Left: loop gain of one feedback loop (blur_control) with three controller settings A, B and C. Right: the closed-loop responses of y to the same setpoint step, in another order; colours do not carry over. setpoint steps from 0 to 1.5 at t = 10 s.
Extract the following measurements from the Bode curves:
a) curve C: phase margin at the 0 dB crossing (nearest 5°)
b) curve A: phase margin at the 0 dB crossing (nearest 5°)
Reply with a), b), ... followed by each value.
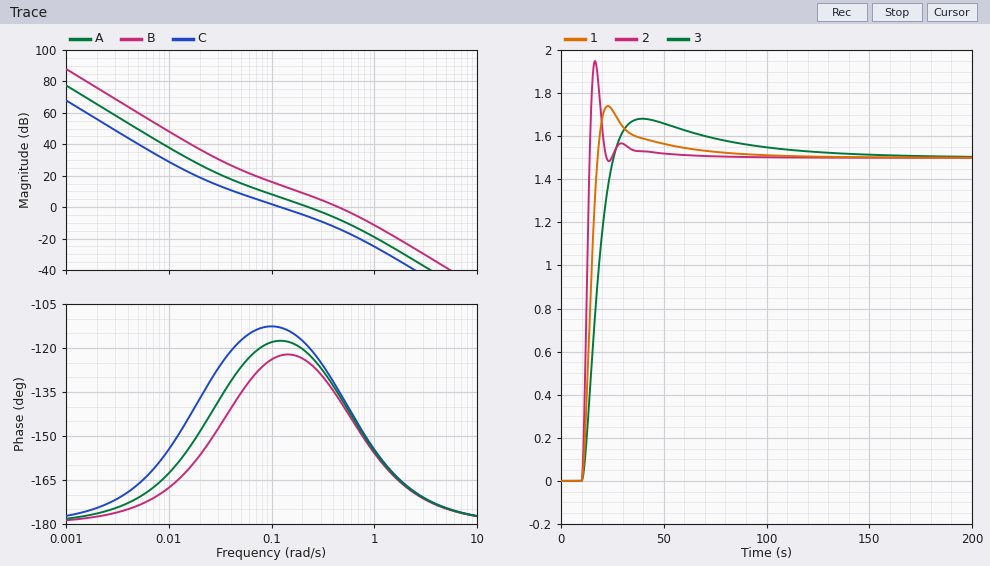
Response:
a) 65°
b) 60°
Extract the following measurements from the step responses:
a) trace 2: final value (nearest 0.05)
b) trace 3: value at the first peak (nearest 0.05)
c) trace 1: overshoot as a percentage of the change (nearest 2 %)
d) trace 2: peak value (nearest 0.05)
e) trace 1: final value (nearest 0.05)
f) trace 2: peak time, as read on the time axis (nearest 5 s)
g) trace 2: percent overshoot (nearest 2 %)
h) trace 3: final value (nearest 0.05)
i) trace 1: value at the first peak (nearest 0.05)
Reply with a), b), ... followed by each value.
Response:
a) 1.50
b) 1.70
c) 16 %
d) 1.95
e) 1.50
f) 15 s
g) 30 %
h) 1.50
i) 1.75
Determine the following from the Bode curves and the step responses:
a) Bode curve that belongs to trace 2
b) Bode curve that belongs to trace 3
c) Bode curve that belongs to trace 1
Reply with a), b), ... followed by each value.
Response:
a) B
b) C
c) A
